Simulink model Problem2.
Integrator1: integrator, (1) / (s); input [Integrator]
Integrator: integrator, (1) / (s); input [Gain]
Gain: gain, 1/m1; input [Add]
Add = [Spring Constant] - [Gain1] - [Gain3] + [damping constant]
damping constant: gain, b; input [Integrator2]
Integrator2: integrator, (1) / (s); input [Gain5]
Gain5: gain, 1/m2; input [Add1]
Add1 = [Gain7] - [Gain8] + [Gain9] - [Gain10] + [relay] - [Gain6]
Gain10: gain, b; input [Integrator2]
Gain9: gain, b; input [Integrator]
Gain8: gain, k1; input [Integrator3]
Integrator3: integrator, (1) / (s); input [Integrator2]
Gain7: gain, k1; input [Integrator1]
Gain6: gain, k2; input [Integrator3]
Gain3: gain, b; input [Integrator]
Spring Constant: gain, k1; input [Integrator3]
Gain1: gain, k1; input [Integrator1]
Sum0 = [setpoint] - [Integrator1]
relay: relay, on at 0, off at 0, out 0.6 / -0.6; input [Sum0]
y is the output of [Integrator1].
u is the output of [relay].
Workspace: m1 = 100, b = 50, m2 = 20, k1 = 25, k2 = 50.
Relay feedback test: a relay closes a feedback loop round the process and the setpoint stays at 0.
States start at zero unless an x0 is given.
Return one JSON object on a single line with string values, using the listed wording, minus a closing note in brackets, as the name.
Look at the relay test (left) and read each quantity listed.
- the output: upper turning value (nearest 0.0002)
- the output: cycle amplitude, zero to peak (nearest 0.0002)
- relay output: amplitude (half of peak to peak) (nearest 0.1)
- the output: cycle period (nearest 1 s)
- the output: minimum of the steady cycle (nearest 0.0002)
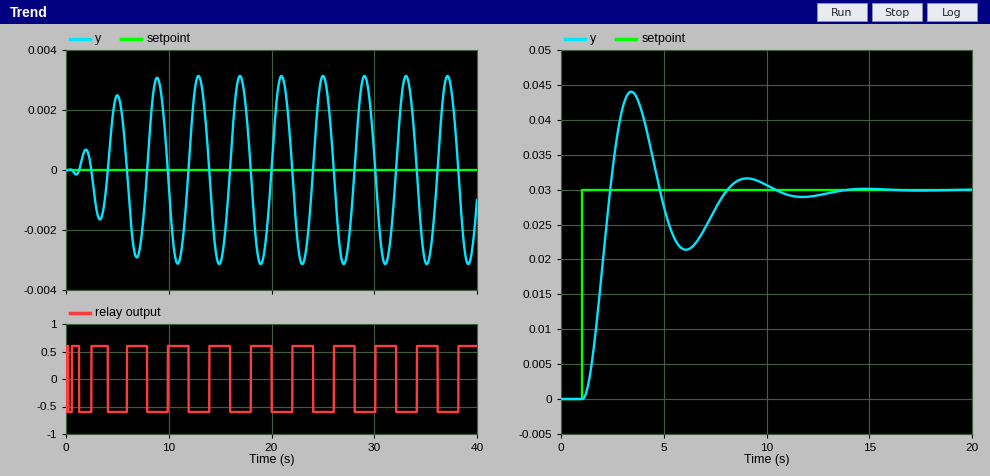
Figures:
{"the output: upper turning value": "0.0032", "the output: cycle amplitude, zero to peak": "0.0032", "relay output: amplitude (half of peak to peak)": "0.6", "the output: cycle period": "4 s", "the output: minimum of the steady cycle": "-0.0032"}
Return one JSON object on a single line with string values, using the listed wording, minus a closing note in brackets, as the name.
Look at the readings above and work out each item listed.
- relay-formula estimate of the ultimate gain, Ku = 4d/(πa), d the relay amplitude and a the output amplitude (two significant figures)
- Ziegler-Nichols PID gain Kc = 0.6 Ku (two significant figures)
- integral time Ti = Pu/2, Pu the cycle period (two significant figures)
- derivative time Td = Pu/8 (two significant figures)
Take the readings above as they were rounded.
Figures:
{"relay-formula estimate of the ultimate gain, Ku = 4d/(πa), d the relay amplitude and a the output amplitude": "240", "Ziegler-Nichols PID gain Kc = 0.6 Ku": "140", "integral time Ti = Pu/2, Pu the cycle period": "2.0 s", "derivative time Td = Pu/8": "0.50 s"}
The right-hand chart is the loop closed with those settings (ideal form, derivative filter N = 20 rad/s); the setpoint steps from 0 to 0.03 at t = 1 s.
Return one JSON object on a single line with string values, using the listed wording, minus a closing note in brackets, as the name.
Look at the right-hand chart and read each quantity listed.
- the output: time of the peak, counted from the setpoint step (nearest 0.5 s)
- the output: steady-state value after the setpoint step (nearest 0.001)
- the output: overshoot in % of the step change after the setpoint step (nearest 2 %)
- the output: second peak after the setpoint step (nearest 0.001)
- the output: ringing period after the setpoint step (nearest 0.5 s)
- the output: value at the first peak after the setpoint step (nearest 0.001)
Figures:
{"the output: time of the peak, counted from the setpoint step": "2.5 s", "the output: steady-state value after the setpoint step": "0.030", "the output: overshoot in % of the step change after the setpoint step": "46 %", "the output: second peak after the setpoint step": "0.032", "the output: ringing period after the setpoint step": "5.5 s", "the output: value at the first peak after the setpoint step": "0.044"}
